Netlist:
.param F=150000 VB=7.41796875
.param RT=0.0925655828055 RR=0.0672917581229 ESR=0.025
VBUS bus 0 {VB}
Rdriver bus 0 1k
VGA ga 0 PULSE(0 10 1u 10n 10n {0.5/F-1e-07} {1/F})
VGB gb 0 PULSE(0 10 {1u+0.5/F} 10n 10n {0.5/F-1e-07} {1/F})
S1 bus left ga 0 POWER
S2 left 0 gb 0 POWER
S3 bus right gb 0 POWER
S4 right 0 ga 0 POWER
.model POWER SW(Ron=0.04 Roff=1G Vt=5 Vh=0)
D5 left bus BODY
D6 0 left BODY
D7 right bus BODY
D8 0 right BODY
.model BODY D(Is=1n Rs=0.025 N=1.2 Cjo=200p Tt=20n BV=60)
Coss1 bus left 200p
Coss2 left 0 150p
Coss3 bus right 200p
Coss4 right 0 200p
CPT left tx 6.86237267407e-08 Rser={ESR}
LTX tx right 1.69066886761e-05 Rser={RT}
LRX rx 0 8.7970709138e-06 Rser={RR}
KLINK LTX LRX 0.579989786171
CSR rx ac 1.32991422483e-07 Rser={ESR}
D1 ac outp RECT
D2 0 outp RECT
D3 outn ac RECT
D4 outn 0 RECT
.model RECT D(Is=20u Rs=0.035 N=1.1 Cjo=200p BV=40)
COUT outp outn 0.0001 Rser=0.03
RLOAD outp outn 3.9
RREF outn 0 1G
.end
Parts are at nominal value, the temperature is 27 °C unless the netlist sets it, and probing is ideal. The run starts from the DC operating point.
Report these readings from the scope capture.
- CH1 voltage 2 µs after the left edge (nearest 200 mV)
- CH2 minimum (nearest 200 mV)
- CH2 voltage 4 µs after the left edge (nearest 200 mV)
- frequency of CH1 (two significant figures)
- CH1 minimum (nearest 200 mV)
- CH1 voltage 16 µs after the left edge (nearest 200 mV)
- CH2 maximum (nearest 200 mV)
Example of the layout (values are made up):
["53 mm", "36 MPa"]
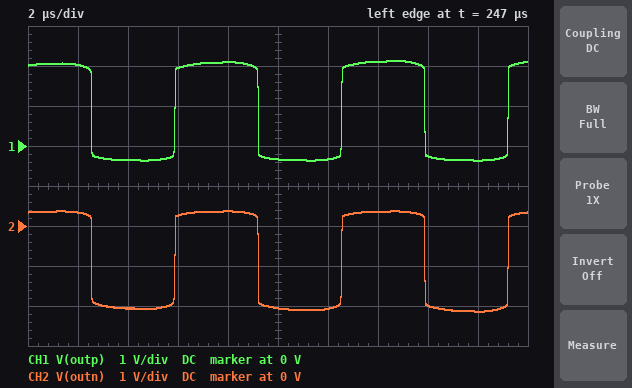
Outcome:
["2.0 V", "-2.2 V", "-2.0 V", "150 kHz", "-400 mV", "-200 mV", "400 mV"]
